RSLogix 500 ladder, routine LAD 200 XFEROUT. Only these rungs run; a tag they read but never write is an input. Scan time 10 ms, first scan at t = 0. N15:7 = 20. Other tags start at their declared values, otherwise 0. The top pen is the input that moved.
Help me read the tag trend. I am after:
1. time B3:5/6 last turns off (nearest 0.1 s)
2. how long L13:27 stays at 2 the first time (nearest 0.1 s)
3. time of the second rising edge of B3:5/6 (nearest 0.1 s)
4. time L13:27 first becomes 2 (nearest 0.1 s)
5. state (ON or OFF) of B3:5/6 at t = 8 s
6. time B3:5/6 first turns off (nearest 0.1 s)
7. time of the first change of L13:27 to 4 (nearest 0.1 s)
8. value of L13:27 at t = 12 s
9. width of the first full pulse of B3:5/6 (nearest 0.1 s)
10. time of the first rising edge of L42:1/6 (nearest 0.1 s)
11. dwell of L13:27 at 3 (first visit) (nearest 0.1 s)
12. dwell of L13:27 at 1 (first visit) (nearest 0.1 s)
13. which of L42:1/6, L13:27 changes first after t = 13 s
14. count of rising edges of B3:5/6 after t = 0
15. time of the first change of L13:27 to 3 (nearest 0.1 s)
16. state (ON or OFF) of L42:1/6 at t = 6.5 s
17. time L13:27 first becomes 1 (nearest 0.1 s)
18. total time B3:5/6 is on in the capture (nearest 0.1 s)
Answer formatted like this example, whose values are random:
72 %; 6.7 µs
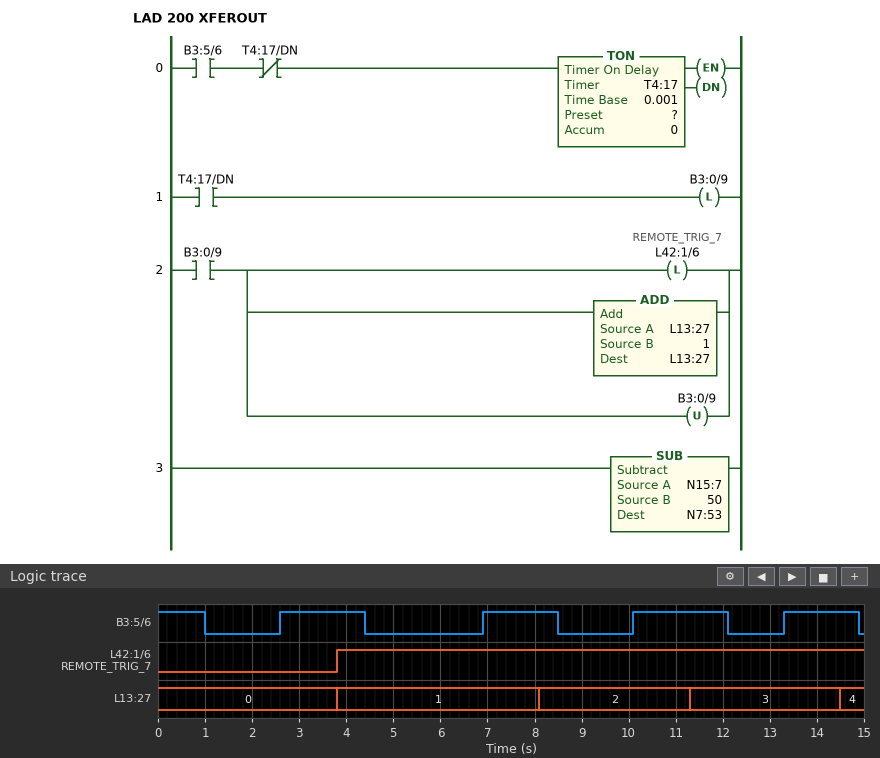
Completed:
14.9 s; 3.2 s; 6.9 s; 8.1 s; ON; 1.0 s; 14.5 s; 3; 1.8 s; 3.8 s; 3.2 s; 4.3 s; L13:27; 4; 11.3 s; ON; 3.8 s; 8.0 s
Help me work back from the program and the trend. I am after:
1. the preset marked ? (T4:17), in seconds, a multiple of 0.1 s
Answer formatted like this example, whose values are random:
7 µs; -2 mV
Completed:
1.2 s
